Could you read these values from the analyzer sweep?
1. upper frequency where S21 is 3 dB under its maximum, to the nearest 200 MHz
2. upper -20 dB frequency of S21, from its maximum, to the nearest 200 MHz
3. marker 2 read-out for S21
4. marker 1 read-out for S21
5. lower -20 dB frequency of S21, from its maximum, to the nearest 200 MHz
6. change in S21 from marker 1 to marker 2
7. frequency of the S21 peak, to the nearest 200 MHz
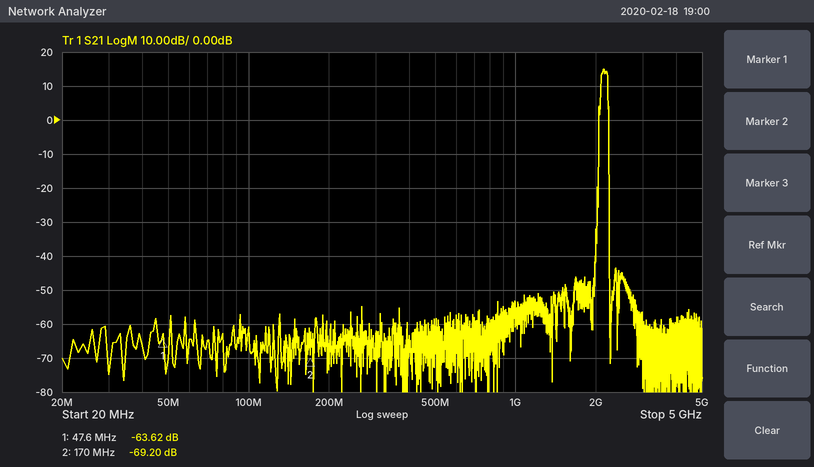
2.2 GHz
2.2 GHz
-69.20 dB
-63.62 dB
2.0 GHz
-5.58 dB
2.2 GHz
